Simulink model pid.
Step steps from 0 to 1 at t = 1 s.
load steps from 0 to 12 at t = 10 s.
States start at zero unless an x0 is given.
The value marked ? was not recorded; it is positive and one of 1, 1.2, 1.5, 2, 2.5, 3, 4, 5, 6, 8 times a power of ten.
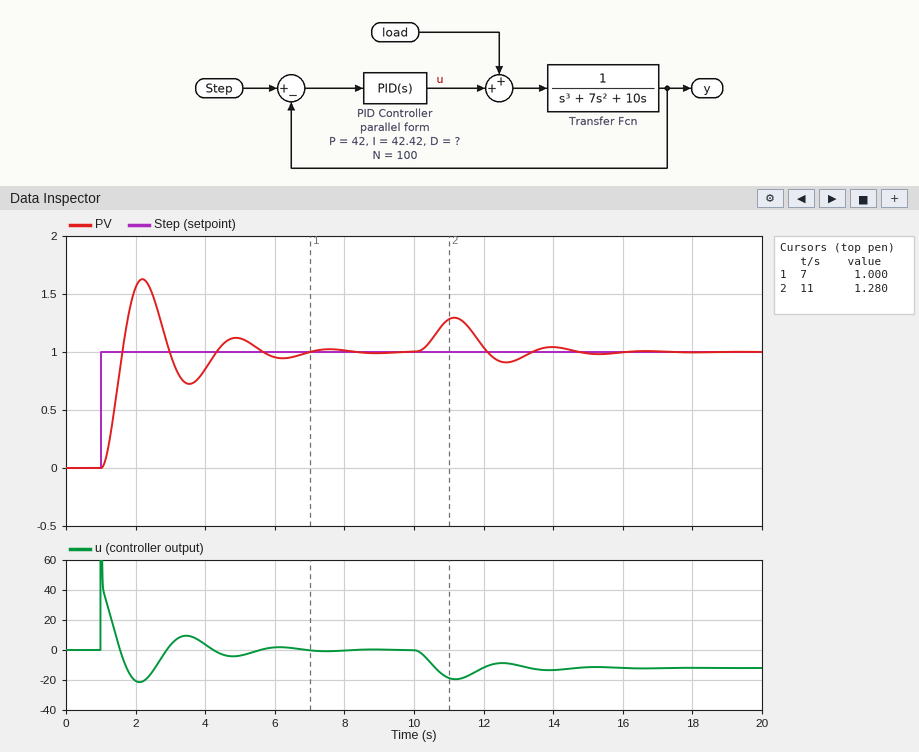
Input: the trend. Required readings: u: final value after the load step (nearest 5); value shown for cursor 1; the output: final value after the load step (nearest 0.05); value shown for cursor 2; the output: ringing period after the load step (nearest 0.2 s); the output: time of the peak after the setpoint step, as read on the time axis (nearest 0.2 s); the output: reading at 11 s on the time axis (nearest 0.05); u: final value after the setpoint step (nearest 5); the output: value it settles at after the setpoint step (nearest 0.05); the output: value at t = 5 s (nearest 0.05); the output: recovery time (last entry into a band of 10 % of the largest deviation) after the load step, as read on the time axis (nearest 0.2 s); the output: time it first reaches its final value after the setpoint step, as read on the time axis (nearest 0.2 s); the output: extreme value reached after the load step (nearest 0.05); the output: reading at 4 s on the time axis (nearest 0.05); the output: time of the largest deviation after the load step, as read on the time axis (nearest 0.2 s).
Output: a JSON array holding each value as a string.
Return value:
["-10", "1.000", "1.00", "1.280", "2.8 s", "2.2 s", "1.30", "0", "1.00", "1.10", "14.4 s", "1.6 s", "1.30", "0.85", "11.2 s"]
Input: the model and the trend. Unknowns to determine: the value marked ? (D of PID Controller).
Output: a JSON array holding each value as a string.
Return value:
["10"]
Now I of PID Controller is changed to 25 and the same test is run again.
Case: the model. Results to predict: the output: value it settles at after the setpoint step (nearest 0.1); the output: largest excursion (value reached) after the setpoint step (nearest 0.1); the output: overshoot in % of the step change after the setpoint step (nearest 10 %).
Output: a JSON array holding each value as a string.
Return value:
["1.0", "1.5", "50 %"]
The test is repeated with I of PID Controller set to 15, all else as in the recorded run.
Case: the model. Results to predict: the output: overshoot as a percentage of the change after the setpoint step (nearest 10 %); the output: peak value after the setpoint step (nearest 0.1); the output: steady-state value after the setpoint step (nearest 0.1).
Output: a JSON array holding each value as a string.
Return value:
["40 %", "1.4", "1.0"]
